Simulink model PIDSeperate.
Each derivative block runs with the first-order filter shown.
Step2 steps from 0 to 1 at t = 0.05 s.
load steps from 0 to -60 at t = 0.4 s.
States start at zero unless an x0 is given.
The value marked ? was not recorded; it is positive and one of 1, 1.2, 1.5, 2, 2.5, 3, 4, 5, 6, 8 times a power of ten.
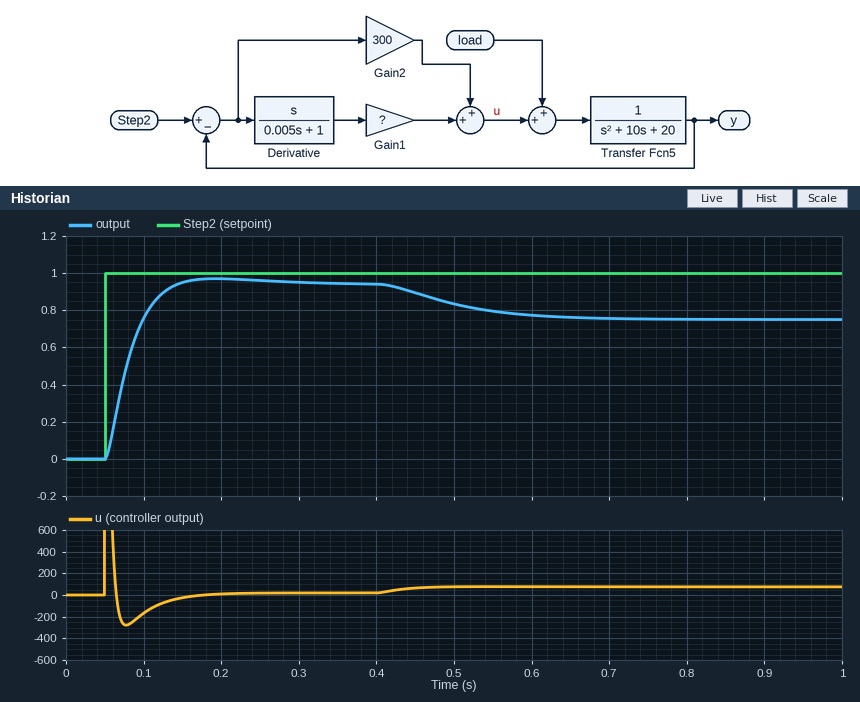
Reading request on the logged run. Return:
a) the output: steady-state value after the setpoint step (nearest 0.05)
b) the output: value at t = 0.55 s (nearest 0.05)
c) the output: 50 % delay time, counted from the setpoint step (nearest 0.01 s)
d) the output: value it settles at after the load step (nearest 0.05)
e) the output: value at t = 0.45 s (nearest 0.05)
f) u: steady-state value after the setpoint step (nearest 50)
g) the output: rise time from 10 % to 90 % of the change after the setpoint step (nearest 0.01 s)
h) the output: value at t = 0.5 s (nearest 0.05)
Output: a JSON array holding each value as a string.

["0.95", "0.80", "0.03 s", "0.75", "0.90", "0", "0.06 s", "0.85"]
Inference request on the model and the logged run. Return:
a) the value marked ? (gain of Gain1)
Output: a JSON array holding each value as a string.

["25"]
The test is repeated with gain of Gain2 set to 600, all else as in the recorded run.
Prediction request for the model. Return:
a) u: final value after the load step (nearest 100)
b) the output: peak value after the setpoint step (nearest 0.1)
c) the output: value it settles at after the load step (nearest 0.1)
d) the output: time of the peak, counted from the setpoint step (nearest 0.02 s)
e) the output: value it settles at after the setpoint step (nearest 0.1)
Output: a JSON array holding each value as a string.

["100", "1.1", "0.9", "0.10 s", "1.0"]
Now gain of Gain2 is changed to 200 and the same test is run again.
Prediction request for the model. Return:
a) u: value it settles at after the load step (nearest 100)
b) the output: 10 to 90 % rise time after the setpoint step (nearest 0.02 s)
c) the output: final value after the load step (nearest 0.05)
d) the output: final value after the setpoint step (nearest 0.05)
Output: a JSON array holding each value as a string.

["100", "0.06 s", "0.65", "0.90"]
